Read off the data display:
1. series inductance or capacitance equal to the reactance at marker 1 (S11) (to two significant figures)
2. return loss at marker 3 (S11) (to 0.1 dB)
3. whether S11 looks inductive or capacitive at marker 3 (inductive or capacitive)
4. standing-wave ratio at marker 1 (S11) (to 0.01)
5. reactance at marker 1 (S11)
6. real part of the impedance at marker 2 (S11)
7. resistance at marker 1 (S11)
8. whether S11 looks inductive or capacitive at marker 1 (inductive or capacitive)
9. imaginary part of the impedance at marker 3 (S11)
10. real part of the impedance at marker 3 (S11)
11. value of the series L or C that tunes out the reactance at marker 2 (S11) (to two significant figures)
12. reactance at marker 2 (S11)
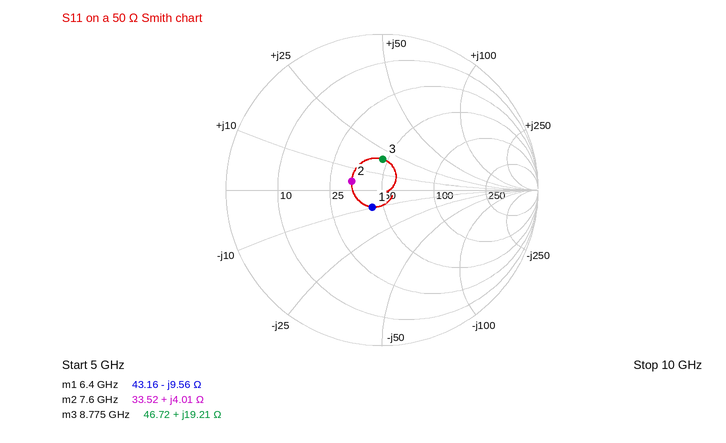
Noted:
2.6 pF
14.1 dB
inductive
1.29
-9.56 Ω
33.52 Ω
43.16 Ω
capacitive
+19.21 Ω
46.72 Ω
5.2 pF
+4.01 Ω
